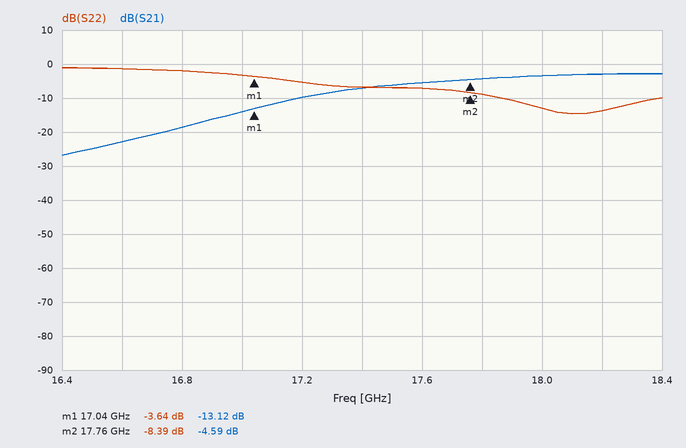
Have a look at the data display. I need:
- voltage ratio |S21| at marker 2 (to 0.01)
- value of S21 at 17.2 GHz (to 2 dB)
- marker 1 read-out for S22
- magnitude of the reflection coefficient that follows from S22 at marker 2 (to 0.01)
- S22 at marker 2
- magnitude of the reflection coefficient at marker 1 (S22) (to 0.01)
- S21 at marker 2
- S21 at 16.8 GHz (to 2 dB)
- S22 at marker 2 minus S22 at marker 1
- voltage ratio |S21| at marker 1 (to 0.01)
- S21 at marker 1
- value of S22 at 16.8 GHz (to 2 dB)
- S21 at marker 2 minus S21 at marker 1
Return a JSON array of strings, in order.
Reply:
["0.59", "-10 dB", "-3.64 dB", "0.38", "-8.39 dB", "0.66", "-4.59 dB", "-18 dB", "-4.75 dB", "0.22", "-13.12 dB", "-2 dB", "8.53 dB"]
